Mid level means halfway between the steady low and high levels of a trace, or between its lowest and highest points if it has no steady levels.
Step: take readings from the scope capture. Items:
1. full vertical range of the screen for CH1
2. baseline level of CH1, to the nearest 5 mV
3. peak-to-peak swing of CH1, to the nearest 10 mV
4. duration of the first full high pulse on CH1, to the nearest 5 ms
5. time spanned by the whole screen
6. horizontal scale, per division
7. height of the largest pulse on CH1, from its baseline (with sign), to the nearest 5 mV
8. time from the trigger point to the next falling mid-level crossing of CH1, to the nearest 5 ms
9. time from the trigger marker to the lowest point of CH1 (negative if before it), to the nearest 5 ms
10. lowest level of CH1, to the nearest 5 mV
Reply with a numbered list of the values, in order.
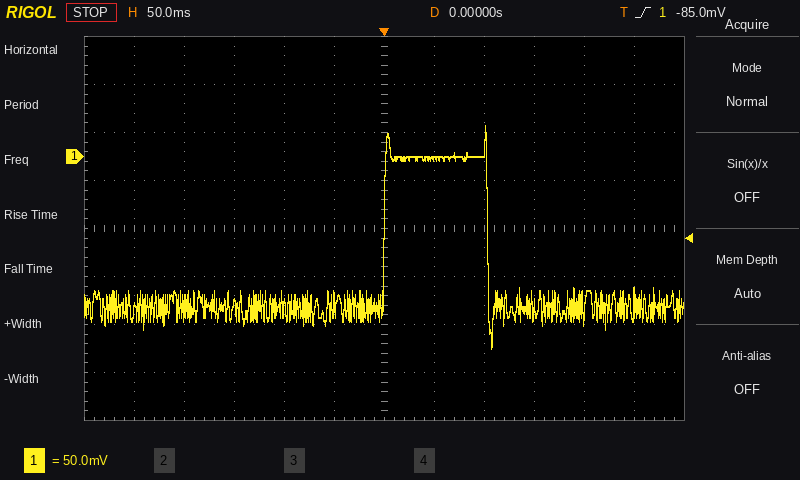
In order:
1. 400 mV
2. -155 mV
3. 230 mV
4. 105 ms
5. 600 ms
6. 50 ms
7. +190 mV
8. 105 ms
9. +110 ms
10. -200 mV
